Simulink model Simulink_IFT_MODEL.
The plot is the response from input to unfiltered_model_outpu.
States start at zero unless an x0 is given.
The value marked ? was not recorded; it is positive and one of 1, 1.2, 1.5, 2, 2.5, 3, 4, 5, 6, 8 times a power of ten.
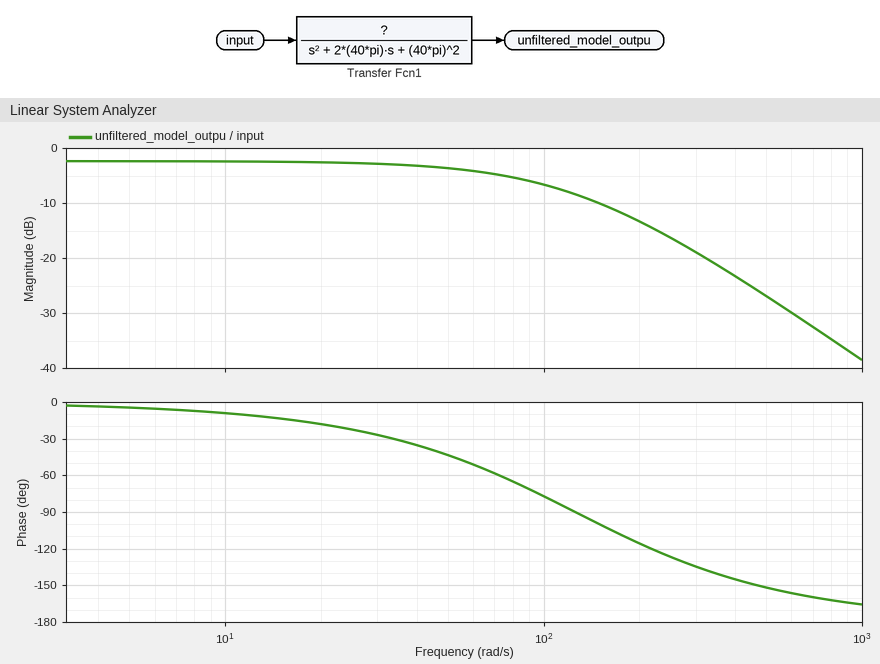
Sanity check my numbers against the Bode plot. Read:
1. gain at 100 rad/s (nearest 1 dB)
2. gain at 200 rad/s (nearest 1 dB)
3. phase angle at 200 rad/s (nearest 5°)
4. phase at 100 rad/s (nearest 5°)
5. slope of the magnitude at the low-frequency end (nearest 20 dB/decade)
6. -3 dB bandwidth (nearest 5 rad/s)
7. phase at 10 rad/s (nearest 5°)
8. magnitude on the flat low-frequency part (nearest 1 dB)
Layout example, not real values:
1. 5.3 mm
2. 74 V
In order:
1. -7 dB
2. -13 dB
3. -115°
4. -75°
5. 0 dB/decade
6. 80 rad/s
7. -10°
8. -2 dB
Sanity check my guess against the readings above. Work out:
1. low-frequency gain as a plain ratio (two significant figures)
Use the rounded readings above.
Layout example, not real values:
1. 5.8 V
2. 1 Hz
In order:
1. 0.79
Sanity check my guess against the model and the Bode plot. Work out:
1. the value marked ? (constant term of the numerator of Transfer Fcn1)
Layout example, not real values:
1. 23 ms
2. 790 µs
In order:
1. 12000
